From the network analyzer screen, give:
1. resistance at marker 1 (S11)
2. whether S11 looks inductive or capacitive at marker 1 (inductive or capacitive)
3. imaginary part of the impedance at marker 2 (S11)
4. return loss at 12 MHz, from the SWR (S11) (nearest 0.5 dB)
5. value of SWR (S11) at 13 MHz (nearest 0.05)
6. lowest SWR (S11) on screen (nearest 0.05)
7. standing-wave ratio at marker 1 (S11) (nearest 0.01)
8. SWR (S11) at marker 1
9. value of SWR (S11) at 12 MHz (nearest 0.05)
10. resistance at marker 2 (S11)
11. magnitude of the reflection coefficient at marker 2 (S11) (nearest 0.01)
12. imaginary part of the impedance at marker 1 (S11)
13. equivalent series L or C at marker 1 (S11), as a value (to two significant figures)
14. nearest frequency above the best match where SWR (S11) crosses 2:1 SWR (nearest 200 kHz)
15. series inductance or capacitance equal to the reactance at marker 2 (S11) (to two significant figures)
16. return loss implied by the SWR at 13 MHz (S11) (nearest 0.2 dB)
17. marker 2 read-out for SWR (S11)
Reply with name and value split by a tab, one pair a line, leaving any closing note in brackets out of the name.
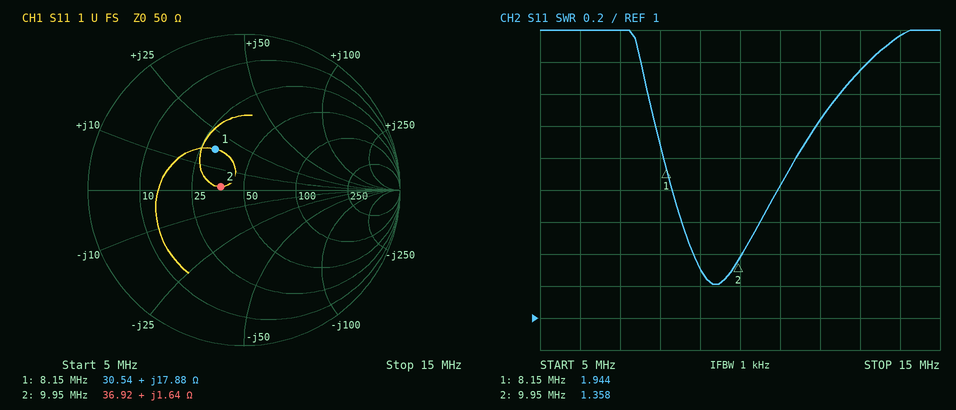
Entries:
resistance at marker 1	30.54 Ω
whether S11 looks inductive or capacitive at marker 1	inductive
imaginary part of the impedance at marker 2	+1.64 Ω
return loss at 12 MHz, from the SWR (S11)	8.5 dB
value of SWR (S11) at 13 MHz	2.55
lowest SWR (S11) on screen	1.20
standing-wave ratio at marker 1 (S11)	1.94
SWR (S11) at marker 1	1.944
value of SWR (S11) at 12 MHz	2.25
resistance at marker 2	36.92 Ω
magnitude of the reflection coefficient at marker 2 (S11)	0.15
imaginary part of the impedance at marker 1	+17.88 Ω
equivalent series L or C at marker 1 (S11), as a value	350 nH
nearest frequency above the best match where SWR (S11) crosses 2:1 SWR	11.4 MHz
series inductance or capacitance equal to the reactance at marker 2 (S11)	26 nH
return loss implied by the SWR at 13 MHz (S11)	7.2 dB
marker 2 read-out for SWR	1.358
